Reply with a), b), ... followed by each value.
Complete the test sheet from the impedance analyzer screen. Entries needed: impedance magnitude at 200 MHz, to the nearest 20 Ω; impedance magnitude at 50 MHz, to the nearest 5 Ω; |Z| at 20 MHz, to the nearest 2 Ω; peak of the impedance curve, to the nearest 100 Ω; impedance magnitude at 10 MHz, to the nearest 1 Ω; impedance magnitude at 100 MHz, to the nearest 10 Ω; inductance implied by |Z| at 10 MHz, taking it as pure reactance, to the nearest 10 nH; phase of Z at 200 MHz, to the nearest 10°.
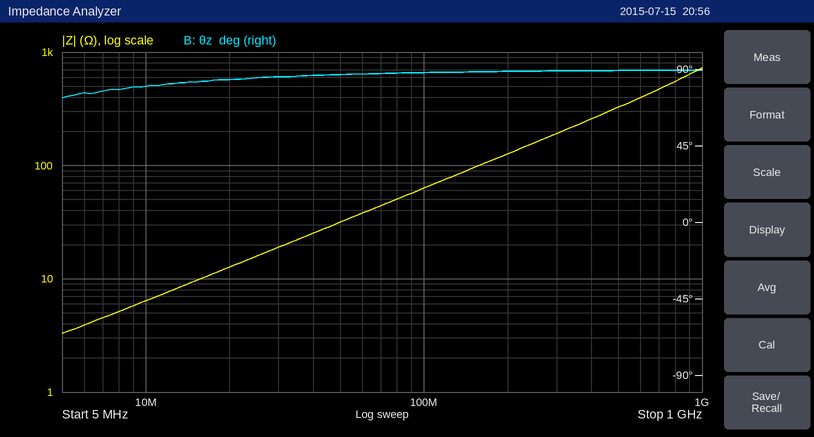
a) 120 Ω
b) 30 Ω
c) 12 Ω
d) 700 Ω
e) 6 Ω
f) 60 Ω
g) 100 nH
h) 90°
